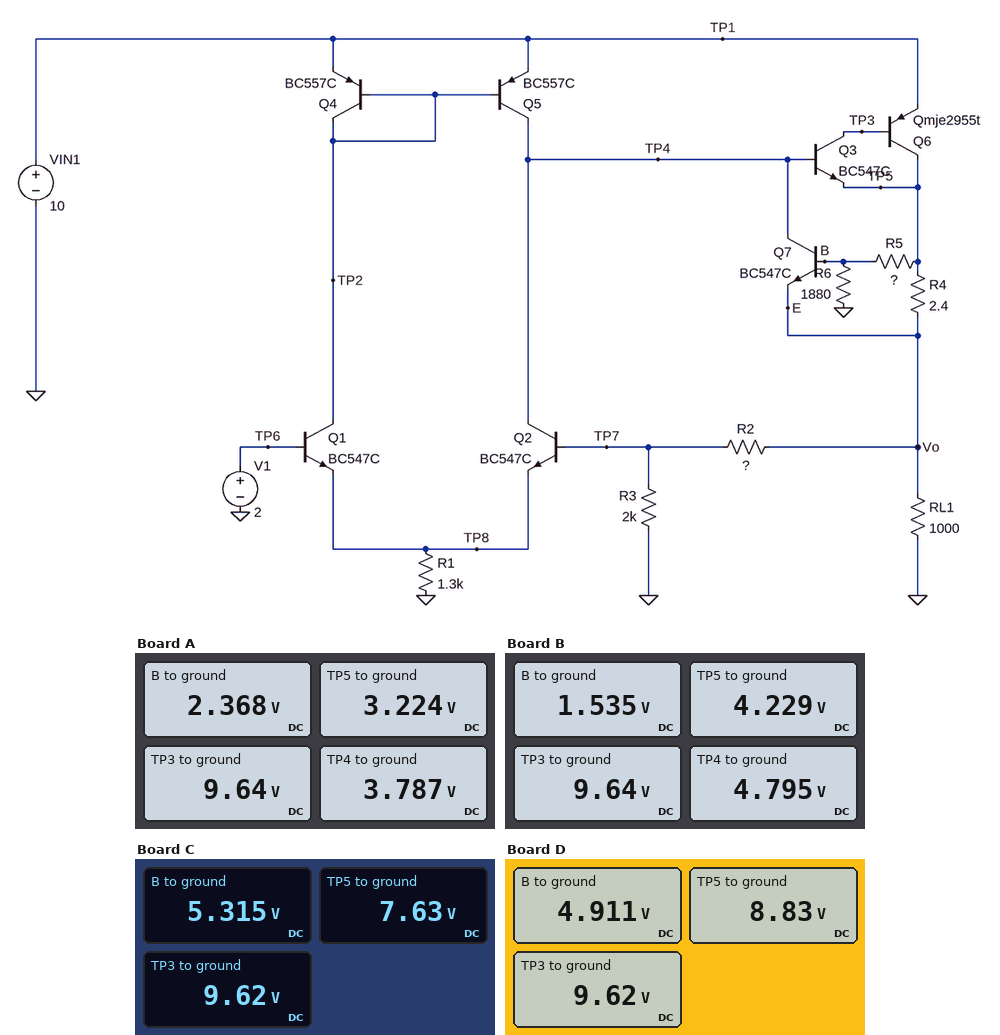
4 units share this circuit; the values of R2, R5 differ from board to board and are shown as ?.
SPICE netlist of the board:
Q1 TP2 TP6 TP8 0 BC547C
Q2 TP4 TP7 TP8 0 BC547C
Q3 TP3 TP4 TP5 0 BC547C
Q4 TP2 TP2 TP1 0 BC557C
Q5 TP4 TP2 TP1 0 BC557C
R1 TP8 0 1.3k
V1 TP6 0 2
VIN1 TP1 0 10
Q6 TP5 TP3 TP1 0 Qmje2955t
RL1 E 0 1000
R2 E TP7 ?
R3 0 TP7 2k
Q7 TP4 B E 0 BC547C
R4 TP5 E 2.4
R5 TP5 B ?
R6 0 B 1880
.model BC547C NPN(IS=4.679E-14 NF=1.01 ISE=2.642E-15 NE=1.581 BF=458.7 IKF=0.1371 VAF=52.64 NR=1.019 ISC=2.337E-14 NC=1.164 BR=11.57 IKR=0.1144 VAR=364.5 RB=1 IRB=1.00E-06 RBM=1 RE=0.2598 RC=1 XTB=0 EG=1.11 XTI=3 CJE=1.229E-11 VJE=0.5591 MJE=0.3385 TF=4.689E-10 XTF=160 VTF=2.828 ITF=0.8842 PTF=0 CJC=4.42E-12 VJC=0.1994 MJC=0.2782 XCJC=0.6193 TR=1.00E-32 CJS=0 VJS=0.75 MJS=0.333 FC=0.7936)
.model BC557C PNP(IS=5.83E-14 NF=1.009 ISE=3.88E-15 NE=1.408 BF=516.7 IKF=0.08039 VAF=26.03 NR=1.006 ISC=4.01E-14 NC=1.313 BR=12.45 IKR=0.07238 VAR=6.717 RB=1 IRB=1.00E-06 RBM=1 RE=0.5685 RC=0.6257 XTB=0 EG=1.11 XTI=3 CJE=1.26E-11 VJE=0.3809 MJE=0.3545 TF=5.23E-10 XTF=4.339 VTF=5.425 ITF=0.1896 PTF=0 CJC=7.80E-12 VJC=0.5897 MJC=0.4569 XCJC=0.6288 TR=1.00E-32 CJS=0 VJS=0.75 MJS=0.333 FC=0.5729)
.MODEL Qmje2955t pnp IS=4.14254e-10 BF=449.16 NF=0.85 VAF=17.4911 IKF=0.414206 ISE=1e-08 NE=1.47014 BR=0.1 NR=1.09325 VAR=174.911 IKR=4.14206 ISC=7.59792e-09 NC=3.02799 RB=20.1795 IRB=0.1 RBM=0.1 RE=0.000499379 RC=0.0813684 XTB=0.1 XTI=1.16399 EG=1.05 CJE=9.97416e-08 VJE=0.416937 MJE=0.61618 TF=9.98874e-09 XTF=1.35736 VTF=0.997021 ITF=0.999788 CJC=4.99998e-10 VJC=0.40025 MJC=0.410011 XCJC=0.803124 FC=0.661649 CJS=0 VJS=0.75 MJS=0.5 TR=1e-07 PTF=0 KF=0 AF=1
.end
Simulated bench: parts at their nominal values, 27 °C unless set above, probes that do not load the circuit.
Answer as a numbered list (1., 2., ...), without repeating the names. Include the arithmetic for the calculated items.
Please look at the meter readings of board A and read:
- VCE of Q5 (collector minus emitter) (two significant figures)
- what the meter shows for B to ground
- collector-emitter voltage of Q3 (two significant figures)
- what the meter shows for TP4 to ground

1. 3.787 V - 10 V = -6.2 V
2. 2.368 V
3. 9.64 V - 3.224 V = 6.4 V
4. 3.787 V
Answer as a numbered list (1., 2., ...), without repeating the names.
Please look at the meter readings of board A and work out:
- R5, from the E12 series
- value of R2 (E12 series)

1. 680 Ω
2. 1.2 kΩ
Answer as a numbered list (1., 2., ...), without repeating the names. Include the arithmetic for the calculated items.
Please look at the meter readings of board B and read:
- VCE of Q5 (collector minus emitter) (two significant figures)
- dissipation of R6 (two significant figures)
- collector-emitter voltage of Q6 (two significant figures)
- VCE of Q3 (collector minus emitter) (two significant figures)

1. 4.795 V - 10 V = -5.2 V
2. (1.535 V)^2 / 1.88 kΩ = 1.3 mW
3. 4.229 V - 10 V = -5.8 V
4. 9.64 V - 4.229 V = 5.4 V
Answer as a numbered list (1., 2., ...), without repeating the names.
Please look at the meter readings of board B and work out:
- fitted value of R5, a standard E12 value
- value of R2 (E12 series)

1. 3.3 kΩ
2. 2.2 kΩ
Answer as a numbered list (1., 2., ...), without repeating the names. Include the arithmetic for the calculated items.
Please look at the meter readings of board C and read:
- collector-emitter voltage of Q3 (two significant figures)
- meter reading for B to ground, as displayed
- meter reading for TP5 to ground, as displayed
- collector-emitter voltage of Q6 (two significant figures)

1. 9.62 V - 7.63 V = 2.0 V
2. 5.315 V
3. 7.63 V
4. 7.63 V - 10 V = -2.4 V
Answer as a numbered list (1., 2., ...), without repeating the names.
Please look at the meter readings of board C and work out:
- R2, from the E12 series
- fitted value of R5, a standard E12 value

1. 5.6 kΩ
2. 820 Ω
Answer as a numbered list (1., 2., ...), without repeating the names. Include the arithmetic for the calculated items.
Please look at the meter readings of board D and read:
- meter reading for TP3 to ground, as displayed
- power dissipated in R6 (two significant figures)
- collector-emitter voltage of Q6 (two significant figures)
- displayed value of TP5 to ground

1. 9.62 V
2. (4.911 V)^2 / 1.88 kΩ = 13 mW
3. 8.83 V - 10 V = -1.2 V
4. 8.83 V
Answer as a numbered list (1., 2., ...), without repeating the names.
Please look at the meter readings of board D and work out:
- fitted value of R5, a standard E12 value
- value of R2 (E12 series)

1. 1.5 kΩ
2. 6.8 kΩ
